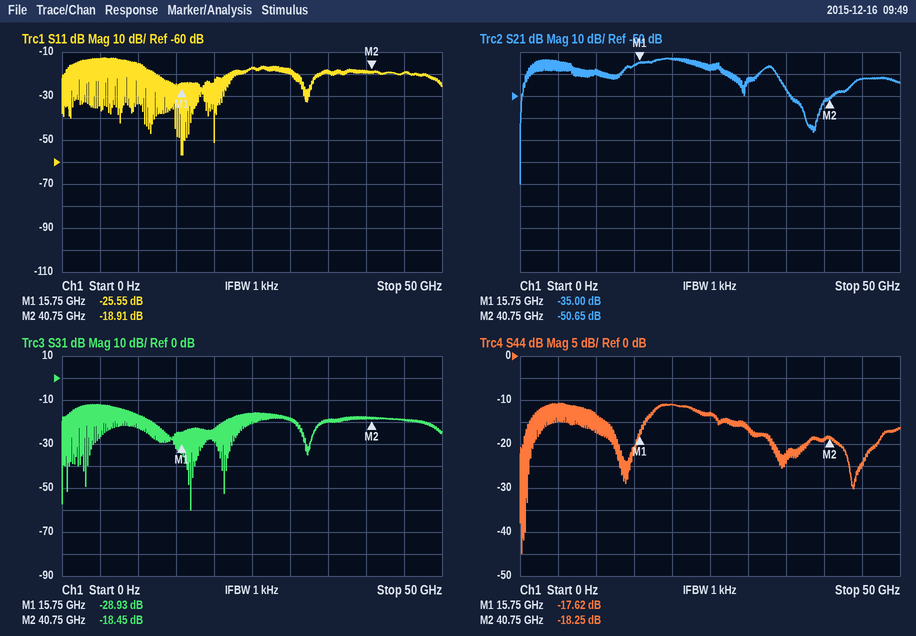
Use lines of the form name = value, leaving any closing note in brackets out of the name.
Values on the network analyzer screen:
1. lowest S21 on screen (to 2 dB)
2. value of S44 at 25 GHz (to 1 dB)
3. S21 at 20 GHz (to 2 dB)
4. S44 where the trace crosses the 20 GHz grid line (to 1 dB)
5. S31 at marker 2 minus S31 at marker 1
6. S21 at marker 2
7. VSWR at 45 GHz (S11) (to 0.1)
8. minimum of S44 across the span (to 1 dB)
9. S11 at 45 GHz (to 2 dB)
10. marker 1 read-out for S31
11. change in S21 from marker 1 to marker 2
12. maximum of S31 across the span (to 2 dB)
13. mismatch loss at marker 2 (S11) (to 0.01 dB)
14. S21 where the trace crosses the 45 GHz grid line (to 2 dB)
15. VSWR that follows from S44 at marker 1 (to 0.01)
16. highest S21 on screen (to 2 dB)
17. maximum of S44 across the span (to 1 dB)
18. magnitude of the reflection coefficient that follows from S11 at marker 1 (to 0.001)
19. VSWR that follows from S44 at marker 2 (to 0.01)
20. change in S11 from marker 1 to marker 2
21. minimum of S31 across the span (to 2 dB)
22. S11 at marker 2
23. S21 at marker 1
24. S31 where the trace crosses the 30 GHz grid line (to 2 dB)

lowest S21 on screen = -90 dB
value of S44 at 25 GHz = -13 dB
S21 at 20 GHz = -34 dB
S44 where the trace crosses the 20 GHz grid line = -11 dB
S31 at marker 2 minus S31 at marker 1 = 10.48 dB
S21 at marker 2 = -50.65 dB
VSWR at 45 GHz (S11) = 1.2
minimum of S44 across the span = -45 dB
S11 at 45 GHz = -20 dB
marker 1 read-out for S31 = -28.93 dB
change in S21 from marker 1 to marker 2 = -15.65 dB
maximum of S31 across the span = -12 dB
mismatch loss at marker 2 (S11) = 0.06 dB
S21 where the trace crosses the 45 GHz grid line = -42 dB
VSWR that follows from S44 at marker 1 = 1.30
highest S21 on screen = -32 dB
maximum of S44 across the span = -11 dB
magnitude of the reflection coefficient that follows from S11 at marker 1 = 0.053
VSWR that follows from S44 at marker 2 = 1.28
change in S11 from marker 1 to marker 2 = 6.64 dB
minimum of S31 across the span = -60 dB
S11 at marker 2 = -18.91 dB
S21 at marker 1 = -35.00 dB
S31 where the trace crosses the 30 GHz grid line = -18 dB
